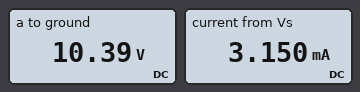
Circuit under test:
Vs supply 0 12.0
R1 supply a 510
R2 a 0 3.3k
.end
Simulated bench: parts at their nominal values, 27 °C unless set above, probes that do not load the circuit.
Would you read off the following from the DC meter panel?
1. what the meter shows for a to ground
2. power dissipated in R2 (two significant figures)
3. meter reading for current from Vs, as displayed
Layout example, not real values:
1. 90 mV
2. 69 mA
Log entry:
1. 10.39 V
2. 33 mW
3. 3.150 mA
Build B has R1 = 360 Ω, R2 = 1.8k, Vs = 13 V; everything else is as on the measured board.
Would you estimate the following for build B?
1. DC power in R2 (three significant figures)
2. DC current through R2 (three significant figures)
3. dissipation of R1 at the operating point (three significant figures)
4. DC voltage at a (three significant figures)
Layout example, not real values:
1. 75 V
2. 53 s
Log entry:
1. 65.2 mW
2. 6.02 mA
3. 13.0 mW
4. 10.8 V
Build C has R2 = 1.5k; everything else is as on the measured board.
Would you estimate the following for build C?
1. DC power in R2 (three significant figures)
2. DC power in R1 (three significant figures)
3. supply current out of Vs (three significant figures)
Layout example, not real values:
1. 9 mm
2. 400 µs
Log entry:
1. 53.5 mW
2. 18.2 mW
3. 5.97 mA
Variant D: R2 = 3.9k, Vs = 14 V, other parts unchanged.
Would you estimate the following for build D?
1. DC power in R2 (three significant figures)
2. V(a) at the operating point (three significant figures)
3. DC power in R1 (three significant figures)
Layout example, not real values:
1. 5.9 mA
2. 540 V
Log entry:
1. 39.3 mW
2. 12.4 V
3. 5.14 mW
